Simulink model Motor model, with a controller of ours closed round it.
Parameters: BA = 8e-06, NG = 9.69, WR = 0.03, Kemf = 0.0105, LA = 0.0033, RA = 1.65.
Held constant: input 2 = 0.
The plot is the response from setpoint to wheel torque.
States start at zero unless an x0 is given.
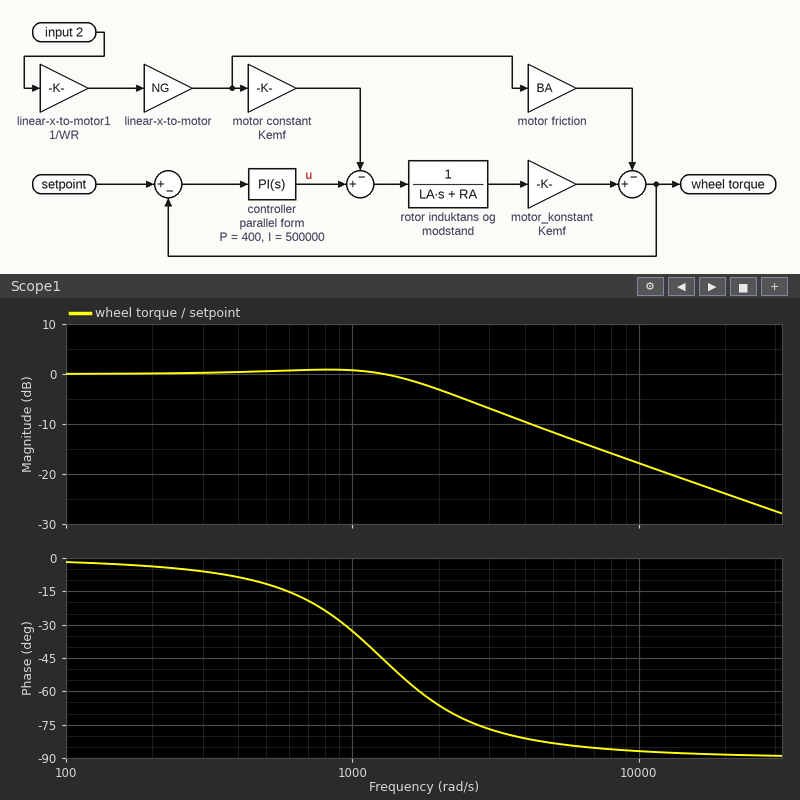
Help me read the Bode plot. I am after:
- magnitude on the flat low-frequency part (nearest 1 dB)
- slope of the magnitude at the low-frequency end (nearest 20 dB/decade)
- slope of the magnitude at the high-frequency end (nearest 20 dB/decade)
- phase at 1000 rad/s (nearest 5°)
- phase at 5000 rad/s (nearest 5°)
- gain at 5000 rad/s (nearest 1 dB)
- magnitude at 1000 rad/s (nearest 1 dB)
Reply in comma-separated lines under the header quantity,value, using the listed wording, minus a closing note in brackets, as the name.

quantity,value
magnitude on the flat low-frequency part,0 dB
slope of the magnitude at the low-frequency end,0 dB/decade
slope of the magnitude at the high-frequency end,-20 dB/decade
phase at 1000 rad/s,-35°
phase at 5000 rad/s,-85°
gain at 5000 rad/s,-12 dB
magnitude at 1000 rad/s,1 dB
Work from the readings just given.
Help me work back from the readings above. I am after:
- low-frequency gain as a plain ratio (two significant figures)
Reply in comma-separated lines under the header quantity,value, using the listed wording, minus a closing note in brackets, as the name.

quantity,value
low-frequency gain as a plain ratio,1.0
